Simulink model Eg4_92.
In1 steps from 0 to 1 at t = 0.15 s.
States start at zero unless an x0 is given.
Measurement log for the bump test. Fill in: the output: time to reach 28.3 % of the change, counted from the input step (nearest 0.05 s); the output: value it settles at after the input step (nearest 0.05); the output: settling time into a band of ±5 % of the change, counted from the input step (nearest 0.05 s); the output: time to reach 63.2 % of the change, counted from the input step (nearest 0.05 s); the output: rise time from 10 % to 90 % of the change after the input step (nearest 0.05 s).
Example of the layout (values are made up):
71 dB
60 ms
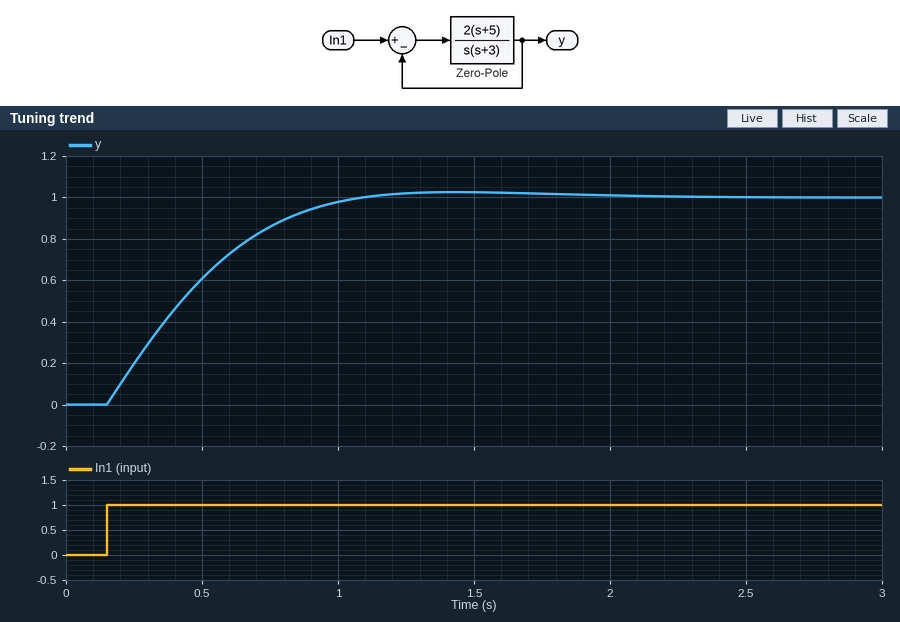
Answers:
0.15 s
1.00
0.75 s
0.35 s
0.60 s
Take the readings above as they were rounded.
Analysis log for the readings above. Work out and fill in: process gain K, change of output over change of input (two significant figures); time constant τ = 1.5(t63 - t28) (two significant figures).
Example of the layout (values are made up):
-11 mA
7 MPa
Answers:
1.0
0.30 s
